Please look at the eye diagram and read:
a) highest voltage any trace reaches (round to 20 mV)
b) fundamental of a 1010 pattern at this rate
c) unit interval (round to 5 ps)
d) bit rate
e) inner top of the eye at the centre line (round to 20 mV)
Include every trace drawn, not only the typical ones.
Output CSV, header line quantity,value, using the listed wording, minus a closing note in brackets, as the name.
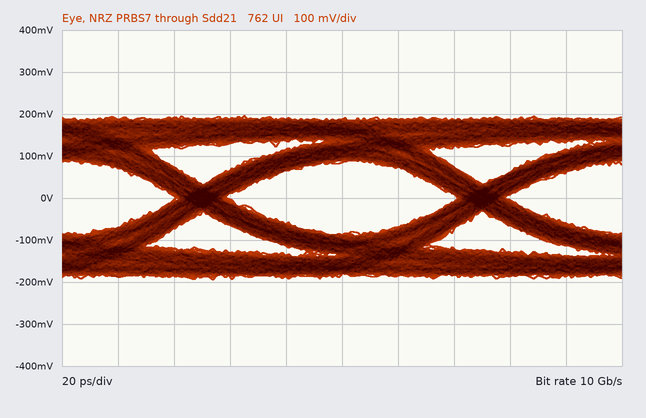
quantity,value
highest voltage any trace reaches,200 mV
fundamental of a 1010 pattern at this rate,5 GHz
unit interval,100 ps
bit rate,10 Gb/s
inner top of the eye at the centre line,80 mV
